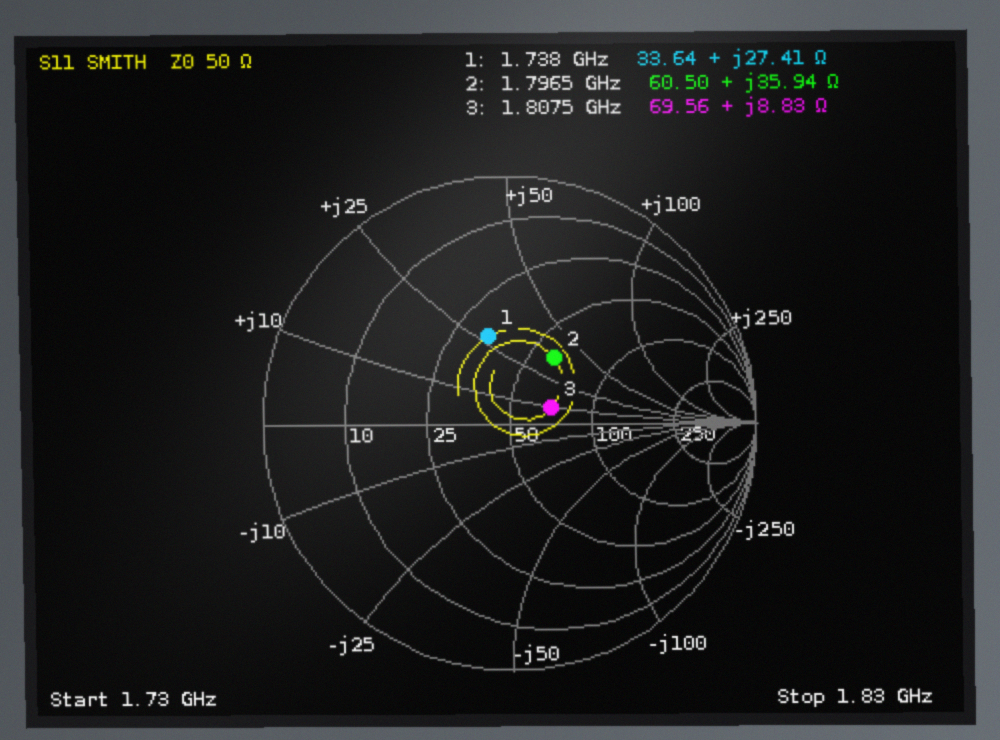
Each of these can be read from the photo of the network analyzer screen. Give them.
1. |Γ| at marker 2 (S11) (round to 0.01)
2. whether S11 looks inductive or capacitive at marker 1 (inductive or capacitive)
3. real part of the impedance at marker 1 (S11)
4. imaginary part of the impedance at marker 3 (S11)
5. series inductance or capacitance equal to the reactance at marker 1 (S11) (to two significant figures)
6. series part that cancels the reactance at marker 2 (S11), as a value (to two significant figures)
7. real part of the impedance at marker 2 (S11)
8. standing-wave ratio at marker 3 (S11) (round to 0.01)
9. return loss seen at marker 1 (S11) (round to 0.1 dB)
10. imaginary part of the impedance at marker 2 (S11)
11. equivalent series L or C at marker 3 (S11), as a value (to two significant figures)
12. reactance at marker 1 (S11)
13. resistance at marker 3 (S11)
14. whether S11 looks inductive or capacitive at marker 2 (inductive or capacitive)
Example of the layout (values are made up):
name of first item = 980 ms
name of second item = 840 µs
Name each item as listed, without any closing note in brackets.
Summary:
|Γ| at marker 2 (S11) = 0.32
whether S11 looks inductive or capacitive at marker 1 = inductive
real part of the impedance at marker 1 = 33.64 Ω
imaginary part of the impedance at marker 3 = +8.83 Ω
series inductance or capacitance equal to the reactance at marker 1 (S11) = 2.5 nH
series part that cancels the reactance at marker 2 (S11), as a value = 2.5 pF
real part of the impedance at marker 2 = 60.50 Ω
standing-wave ratio at marker 3 (S11) = 1.44
return loss seen at marker 1 (S11) = 8.8 dB
imaginary part of the impedance at marker 2 = +35.94 Ω
equivalent series L or C at marker 3 (S11), as a value = 780 pH
reactance at marker 1 = +27.41 Ω
resistance at marker 3 = 69.56 Ω
whether S11 looks inductive or capacitive at marker 2 = inductive
